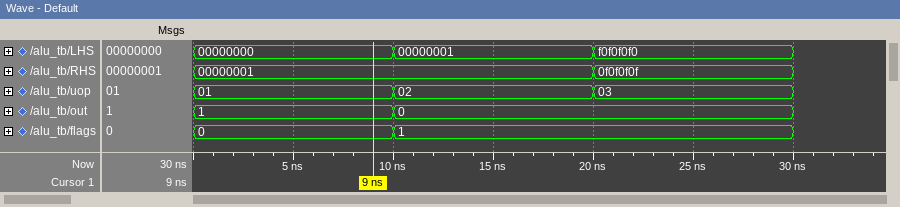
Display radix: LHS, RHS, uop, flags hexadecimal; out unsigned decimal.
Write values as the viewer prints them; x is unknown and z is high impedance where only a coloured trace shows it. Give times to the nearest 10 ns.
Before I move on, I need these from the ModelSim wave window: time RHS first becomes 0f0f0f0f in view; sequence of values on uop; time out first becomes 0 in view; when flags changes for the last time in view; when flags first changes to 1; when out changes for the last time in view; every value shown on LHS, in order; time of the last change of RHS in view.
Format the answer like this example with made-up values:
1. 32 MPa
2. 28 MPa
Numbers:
1. 20 ns
2. 01, 02, 03
3. 10 ns
4. 10 ns
5. 10 ns
6. 10 ns
7. 00000000, 00000001, f0f0f0f0
8. 20 ns
